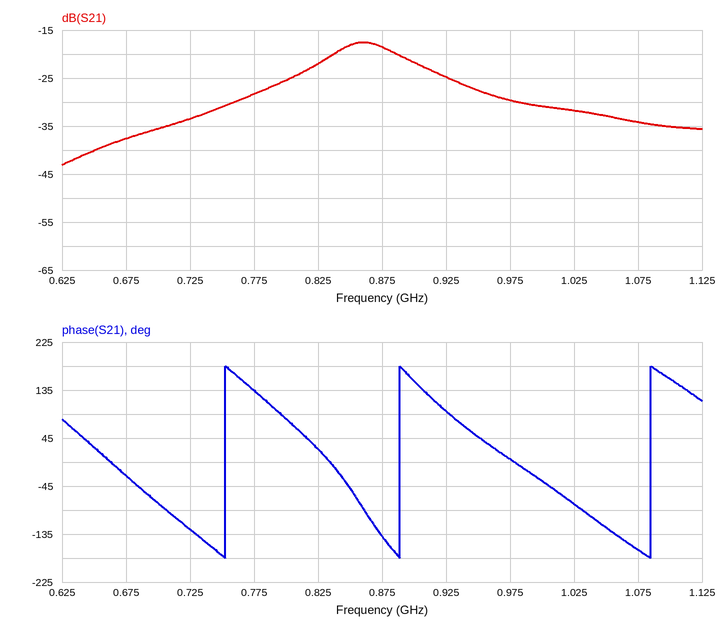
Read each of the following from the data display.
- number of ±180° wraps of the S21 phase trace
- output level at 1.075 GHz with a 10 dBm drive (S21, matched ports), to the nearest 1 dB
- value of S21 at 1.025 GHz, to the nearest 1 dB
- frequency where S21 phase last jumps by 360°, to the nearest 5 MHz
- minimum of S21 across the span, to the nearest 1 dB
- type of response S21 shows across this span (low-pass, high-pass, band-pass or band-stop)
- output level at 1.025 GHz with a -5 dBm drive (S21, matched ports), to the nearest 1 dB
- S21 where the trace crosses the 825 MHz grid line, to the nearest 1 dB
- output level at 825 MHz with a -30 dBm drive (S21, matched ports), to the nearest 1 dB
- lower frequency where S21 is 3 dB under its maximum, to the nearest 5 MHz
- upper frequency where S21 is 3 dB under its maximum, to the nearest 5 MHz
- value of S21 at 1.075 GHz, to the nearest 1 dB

3
-24 dBm
-32 dB
1.085 GHz
-43 dB
band-pass
-37 dBm
-22 dB
-52 dBm
835 MHz
890 MHz
-34 dB
